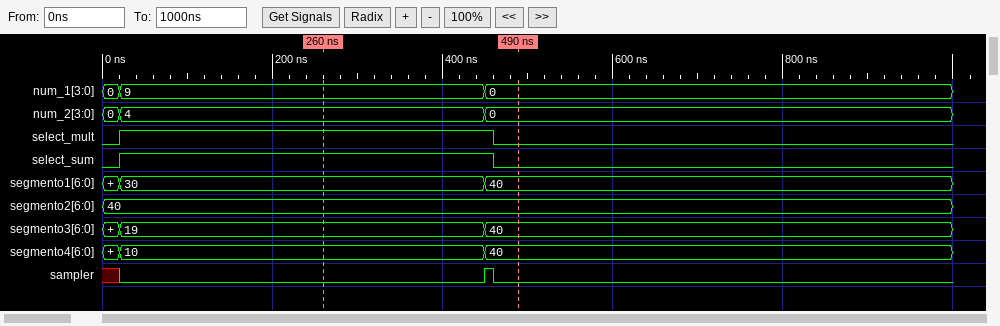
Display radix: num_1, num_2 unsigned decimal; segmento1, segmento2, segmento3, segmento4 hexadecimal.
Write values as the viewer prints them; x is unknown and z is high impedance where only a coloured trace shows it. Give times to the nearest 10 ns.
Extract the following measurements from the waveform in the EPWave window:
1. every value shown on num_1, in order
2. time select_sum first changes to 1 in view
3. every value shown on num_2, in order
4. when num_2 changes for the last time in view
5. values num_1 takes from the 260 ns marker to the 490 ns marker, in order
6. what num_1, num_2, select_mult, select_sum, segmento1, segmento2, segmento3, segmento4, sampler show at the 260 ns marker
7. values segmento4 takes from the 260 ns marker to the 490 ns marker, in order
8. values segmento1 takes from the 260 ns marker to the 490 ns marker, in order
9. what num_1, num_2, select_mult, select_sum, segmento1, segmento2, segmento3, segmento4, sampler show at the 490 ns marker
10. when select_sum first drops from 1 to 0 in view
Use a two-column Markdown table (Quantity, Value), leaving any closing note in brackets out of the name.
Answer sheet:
| Quantity | Value |
|---|---|
| every value shown on num_1, in order | 0, 9, 0 |
| time select_sum first changes to 1 in view | 20 ns |
| every value shown on num_2, in order | 0, 4, 0 |
| when num_2 changes for the last time in view | 450 ns |
| values num_1 takes from the 260 ns marker to the 490 ns marker, in order | 9, 0 |
| what num_1, num_2, select_mult, select_sum, segmento1, segmento2, segmento3, segmento4, sampler show at the 260 ns marker | num_1=9, num_2=4, select_mult=1, select_sum=1, segmento1=30, segmento2=40, segmento3=19, segmento4=10, sampler=0 |
| values segmento4 takes from the 260 ns marker to the 490 ns marker, in order | 10, 40 |
| values segmento1 takes from the 260 ns marker to the 490 ns marker, in order | 30, 40 |
| what num_1, num_2, select_mult, select_sum, segmento1, segmento2, segmento3, segmento4, sampler show at the 490 ns marker | num_1=0, num_2=0, select_mult=0, select_sum=0, segmento1=40, segmento2=40, segmento3=40, segmento4=40, sampler=0 |
| when select_sum first drops from 1 to 0 in view | 460 ns |
